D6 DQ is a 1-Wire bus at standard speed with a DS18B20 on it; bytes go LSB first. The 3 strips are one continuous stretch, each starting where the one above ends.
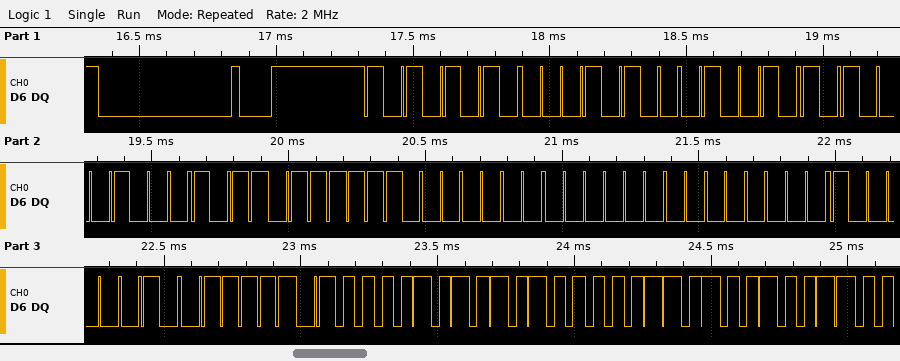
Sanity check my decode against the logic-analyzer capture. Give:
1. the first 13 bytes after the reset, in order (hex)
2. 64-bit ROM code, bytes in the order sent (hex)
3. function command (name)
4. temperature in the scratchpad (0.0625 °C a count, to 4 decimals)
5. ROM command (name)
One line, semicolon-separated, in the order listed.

55 28 52 11 ED 07 00 00 41 BE 50 05 4B; 28 52 11 ED 07 00 00 41; Read Scratchpad; 85.0000 °C; Match ROM
